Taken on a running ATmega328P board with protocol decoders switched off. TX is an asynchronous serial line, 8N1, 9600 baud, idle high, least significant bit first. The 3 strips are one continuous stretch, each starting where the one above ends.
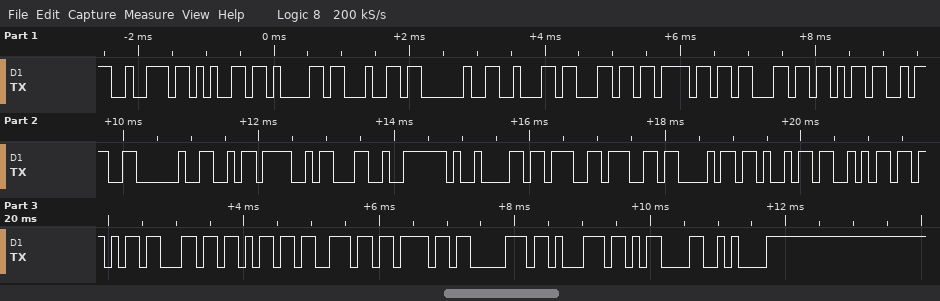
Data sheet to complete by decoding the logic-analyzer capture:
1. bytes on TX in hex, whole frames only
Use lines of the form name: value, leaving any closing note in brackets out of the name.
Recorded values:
bytes on TX in hex, whole frames only: 72 65 61 64 20 62 6C 6F 63 6B 3A 20 DA 1A F2 09 3B 67 68 69 6A 6B 6C 6D 6E 6F 70 71 0D 0A
